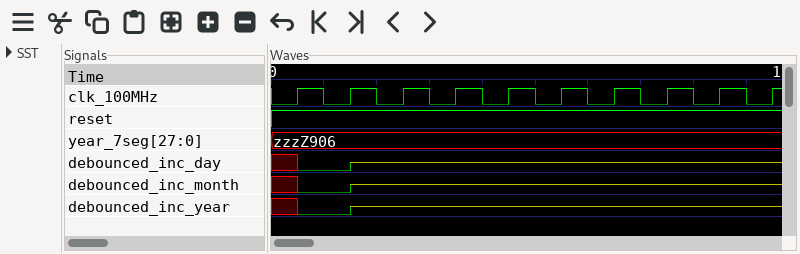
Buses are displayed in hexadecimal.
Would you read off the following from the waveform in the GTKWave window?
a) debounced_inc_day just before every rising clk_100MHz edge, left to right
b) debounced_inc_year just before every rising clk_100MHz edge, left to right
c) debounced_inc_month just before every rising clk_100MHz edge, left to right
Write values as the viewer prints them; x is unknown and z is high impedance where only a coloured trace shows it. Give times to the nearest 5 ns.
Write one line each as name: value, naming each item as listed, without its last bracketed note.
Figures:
debounced_inc_day just before every rising clk_100MHz edge, left to right: x 0 z z z z z z z z
debounced_inc_year just before every rising clk_100MHz edge, left to right: x 0 z z z z z z z z
debounced_inc_month just before every rising clk_100MHz edge, left to right: x 0 z z z z z z z z
